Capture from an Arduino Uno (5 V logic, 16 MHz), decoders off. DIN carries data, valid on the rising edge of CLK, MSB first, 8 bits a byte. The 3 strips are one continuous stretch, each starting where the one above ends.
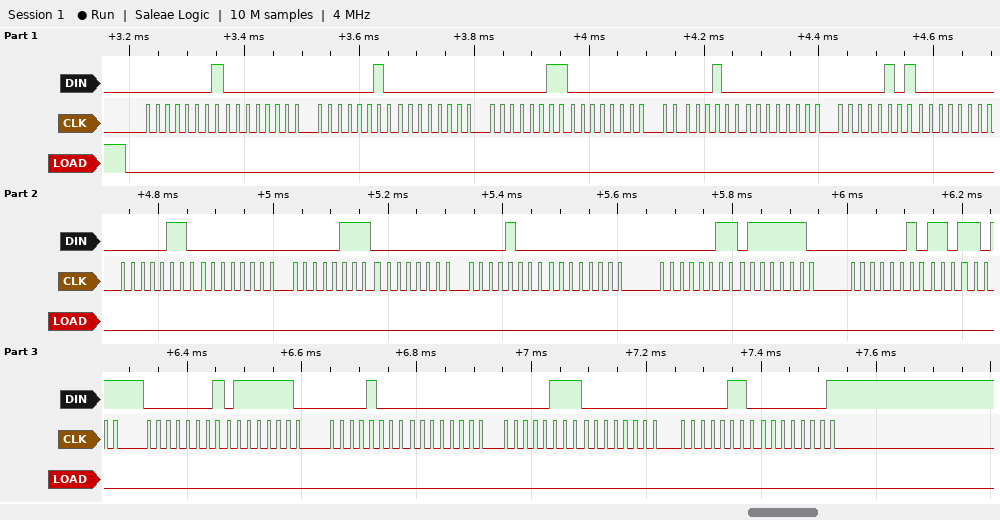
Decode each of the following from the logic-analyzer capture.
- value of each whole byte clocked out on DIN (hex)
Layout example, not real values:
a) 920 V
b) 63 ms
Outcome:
a) 01 00 02 00 03 00 04 00 05 00 06 00 07 00 08 00 03 7E 02 DB 01 7E 08 00 07 00 06 01
